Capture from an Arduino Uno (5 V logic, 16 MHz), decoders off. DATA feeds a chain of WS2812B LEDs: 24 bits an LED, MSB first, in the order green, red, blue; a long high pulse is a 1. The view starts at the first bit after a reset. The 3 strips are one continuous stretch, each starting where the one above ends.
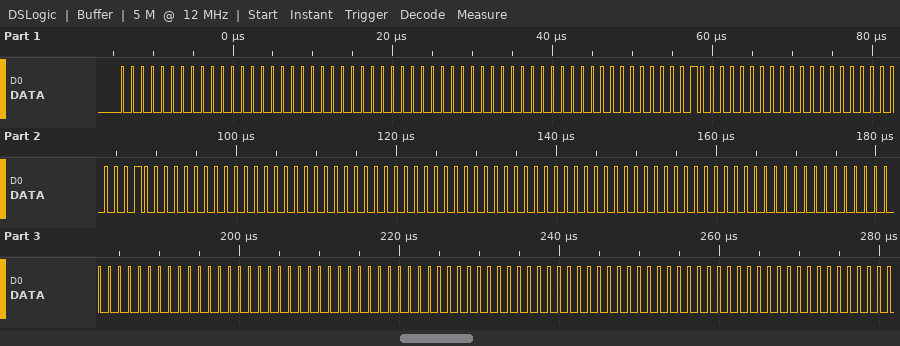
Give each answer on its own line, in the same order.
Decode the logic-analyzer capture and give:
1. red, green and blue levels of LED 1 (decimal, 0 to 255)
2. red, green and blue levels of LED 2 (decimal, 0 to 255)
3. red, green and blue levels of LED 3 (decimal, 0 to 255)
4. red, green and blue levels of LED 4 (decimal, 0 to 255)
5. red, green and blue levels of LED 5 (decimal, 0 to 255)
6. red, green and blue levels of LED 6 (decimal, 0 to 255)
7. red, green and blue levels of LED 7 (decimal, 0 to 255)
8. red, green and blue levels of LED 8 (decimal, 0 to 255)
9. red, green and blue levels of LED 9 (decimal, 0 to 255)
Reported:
0, 0, 0
0, 0, 0
64, 0, 0
64, 0, 0
0, 0, 0
0, 0, 0
0, 0, 0
0, 0, 0
0, 0, 0
